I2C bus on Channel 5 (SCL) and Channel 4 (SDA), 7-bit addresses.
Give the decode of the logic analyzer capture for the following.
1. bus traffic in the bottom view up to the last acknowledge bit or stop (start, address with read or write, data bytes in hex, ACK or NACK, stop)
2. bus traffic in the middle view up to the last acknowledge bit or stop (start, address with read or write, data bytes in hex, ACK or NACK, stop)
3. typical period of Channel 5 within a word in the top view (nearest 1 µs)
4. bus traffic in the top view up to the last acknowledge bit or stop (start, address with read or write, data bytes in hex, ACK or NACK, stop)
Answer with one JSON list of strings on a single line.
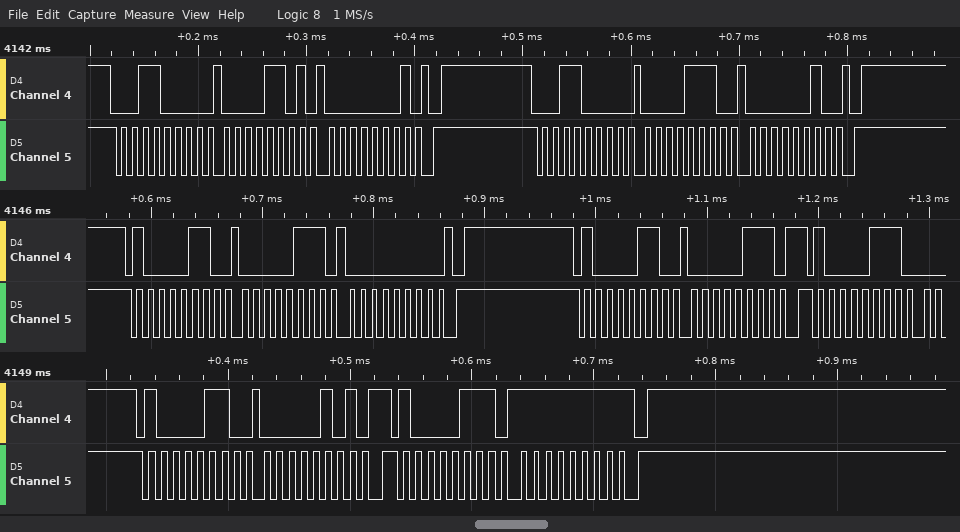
["start, address 43 write ACK, 05 ACK, repeated start, address 43 read ACK, FF NACK, stop", "start, address 43 write ACK, 07 ACK, 00 ACK, stop, start, address 43 write ACK, 07 ACK, repeated start, address 43 read ACK", "10 µs", "start, address 18 write ACK, 0D ACK, 01 ACK, stop, start, address 18 write ACK, 0E ACK, 02 ACK, stop"]
